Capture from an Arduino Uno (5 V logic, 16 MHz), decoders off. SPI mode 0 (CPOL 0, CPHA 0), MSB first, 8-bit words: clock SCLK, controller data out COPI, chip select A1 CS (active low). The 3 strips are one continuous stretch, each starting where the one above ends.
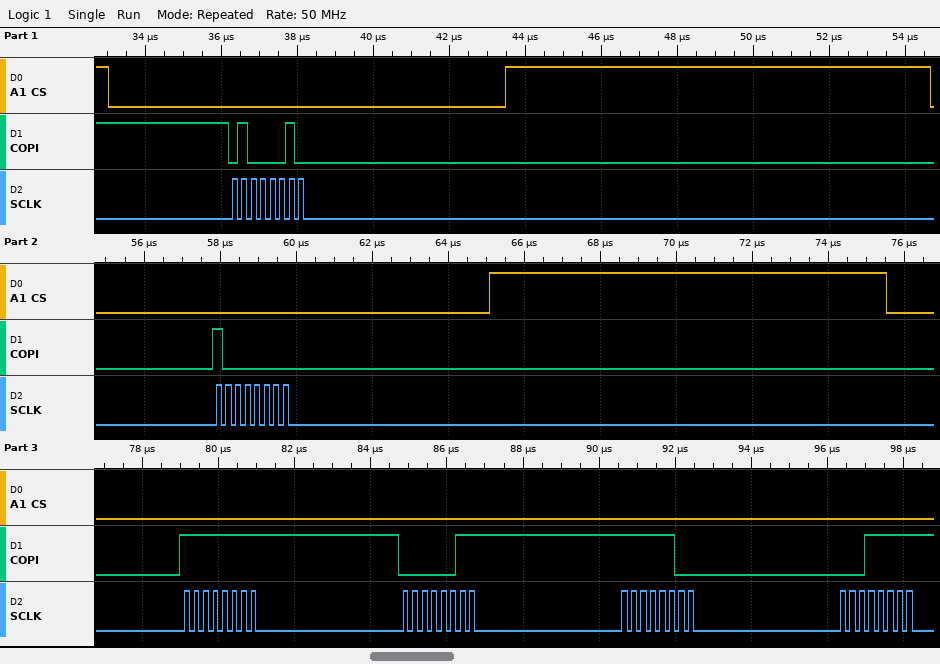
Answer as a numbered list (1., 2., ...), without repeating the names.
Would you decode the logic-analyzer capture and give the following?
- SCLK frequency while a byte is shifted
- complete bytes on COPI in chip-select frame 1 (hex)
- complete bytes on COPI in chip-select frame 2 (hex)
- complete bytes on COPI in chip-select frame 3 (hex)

1. 4 MHz
2. 42
3. 80
4. FF 03 FC 1F
